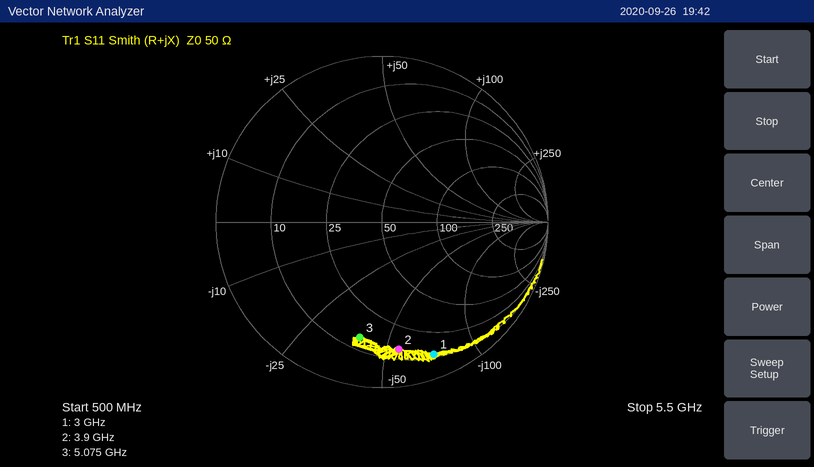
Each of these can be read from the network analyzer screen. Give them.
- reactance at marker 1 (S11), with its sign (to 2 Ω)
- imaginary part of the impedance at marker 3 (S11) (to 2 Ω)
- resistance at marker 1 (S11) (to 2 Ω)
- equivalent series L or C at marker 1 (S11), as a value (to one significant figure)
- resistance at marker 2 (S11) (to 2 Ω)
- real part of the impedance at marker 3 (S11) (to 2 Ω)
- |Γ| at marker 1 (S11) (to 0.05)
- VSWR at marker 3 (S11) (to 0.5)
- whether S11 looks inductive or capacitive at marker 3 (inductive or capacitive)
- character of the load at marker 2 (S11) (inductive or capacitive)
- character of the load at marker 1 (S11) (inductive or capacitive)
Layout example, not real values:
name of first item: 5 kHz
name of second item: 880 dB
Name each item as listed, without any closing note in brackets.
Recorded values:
reactance at marker 1 (S11), with its sign: -72 Ω
imaginary part of the impedance at marker 3 (S11): -40 Ω
resistance at marker 1 (S11): 12 Ω
equivalent series L or C at marker 1 (S11), as a value: 700 fF
resistance at marker 2 (S11): 14 Ω
real part of the impedance at marker 3 (S11): 14 Ω
|Γ| at marker 1 (S11): 0.85
VSWR at marker 3 (S11): 6.0
whether S11 looks inductive or capacitive at marker 3: capacitive
character of the load at marker 2 (S11): capacitive
character of the load at marker 1 (S11): capacitive
